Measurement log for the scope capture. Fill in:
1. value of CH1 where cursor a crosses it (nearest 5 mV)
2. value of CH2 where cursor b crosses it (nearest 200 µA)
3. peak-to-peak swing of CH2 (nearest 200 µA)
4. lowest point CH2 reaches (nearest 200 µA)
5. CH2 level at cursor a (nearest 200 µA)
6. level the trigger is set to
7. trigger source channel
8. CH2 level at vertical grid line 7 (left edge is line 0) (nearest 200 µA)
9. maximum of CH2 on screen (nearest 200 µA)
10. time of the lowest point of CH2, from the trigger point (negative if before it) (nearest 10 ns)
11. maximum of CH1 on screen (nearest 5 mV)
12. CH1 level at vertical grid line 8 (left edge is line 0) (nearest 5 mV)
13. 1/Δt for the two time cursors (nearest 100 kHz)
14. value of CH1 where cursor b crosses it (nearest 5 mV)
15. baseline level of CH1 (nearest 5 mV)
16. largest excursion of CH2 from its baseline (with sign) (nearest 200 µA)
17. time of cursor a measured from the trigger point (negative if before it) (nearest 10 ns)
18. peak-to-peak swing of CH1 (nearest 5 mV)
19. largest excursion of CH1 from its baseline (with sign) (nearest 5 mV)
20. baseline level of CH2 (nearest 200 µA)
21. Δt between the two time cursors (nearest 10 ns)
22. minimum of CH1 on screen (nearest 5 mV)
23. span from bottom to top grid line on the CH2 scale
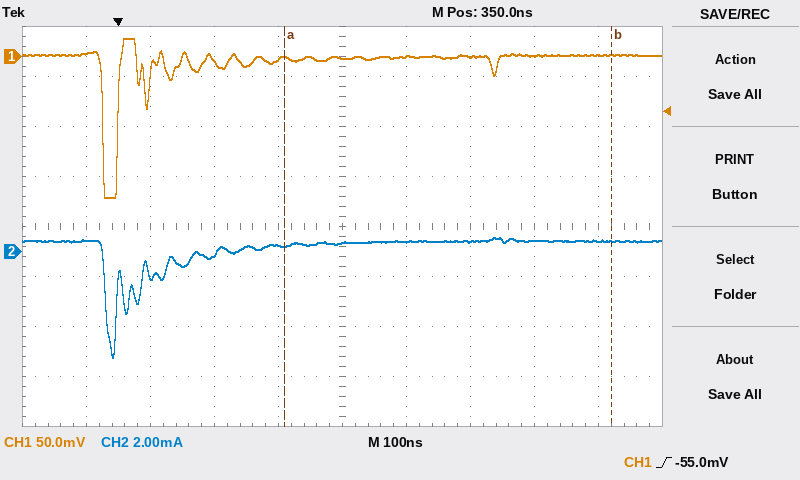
0 mV
400 µA
4.8 mA
-4.2 mA
200 µA
-55.0 mV
CH1
400 µA
600 µA
-10 ns
20 mV
0 mV
2.0 MHz
0 mV
0 mV
-4.6 mA
+260 ns
160 mV
-140 mV
400 µA
510 ns
-140 mV
16 mA
